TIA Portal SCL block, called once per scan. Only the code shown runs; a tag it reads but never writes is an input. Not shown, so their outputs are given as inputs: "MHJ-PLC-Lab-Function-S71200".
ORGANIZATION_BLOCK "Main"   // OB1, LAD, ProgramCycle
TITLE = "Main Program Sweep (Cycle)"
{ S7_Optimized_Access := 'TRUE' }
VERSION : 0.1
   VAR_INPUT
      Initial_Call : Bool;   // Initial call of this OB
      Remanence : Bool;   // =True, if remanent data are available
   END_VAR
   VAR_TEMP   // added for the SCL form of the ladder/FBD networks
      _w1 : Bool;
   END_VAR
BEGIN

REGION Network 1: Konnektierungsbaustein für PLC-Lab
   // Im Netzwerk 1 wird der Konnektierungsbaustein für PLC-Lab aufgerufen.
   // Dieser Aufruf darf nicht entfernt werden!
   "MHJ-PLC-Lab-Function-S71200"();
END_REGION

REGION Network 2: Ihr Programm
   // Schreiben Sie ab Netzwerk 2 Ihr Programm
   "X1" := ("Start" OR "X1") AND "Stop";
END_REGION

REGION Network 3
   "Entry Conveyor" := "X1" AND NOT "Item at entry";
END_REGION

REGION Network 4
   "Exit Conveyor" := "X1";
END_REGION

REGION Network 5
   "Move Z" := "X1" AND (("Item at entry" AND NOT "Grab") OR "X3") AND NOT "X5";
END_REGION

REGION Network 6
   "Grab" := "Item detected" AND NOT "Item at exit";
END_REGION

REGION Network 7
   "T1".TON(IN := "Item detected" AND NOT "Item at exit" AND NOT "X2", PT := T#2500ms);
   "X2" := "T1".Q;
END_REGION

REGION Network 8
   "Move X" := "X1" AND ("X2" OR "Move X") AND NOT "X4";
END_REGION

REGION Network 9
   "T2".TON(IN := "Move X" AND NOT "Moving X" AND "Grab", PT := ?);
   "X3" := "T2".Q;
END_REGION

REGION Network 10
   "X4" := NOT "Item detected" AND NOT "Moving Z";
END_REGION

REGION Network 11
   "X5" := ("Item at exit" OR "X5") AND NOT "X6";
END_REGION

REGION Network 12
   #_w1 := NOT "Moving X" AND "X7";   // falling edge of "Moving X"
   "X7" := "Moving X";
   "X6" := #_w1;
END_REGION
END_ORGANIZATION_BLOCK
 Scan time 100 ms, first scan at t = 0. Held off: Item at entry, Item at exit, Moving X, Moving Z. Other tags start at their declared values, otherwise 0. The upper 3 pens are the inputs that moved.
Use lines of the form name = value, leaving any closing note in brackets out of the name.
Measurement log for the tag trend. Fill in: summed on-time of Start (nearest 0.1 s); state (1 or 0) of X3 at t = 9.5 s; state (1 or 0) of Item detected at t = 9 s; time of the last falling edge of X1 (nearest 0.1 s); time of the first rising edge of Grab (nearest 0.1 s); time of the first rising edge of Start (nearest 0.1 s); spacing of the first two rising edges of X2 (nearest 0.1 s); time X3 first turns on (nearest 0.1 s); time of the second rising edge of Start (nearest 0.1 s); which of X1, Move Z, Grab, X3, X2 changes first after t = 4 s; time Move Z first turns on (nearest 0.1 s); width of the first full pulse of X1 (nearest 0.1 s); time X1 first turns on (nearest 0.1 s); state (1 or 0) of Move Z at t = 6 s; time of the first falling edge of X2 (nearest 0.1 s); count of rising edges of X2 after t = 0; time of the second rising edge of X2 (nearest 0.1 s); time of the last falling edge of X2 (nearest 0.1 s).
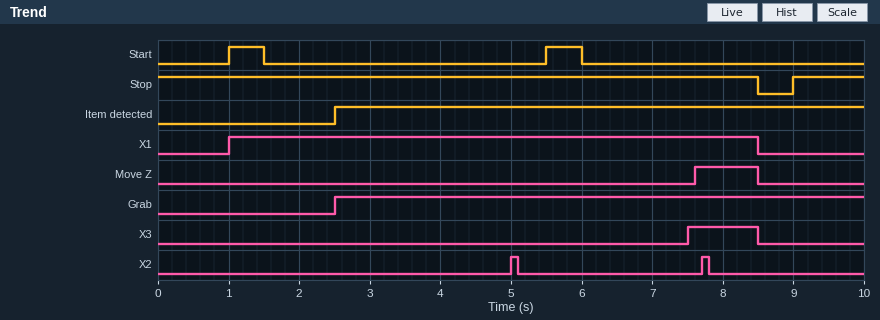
summed on-time of Start = 1.0 s
state (1 or 0) of X3 at t = 9.5 s = 0
state (1 or 0) of Item detected at t = 9 s = 1
time of the last falling edge of X1 = 8.5 s
time of the first rising edge of Grab = 2.5 s
time of the first rising edge of Start = 1.0 s
spacing of the first two rising edges of X2 = 2.7 s
time X3 first turns on = 7.5 s
time of the second rising edge of Start = 5.5 s
which of X1, Move Z, Grab, X3, X2 changes first after t = 4 s = X2
time Move Z first turns on = 7.6 s
width of the first full pulse of X1 = 7.5 s
time X1 first turns on = 1.0 s
state (1 or 0) of Move Z at t = 6 s = 0
time of the first falling edge of X2 = 5.1 s
count of rising edges of X2 after t = 0 = 2
time of the second rising edge of X2 = 7.7 s
time of the last falling edge of X2 = 7.8 s
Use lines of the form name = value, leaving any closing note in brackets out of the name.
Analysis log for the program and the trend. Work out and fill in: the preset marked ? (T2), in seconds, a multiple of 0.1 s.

the preset marked ? (T2), in seconds, a multiple of 0.1 s = 2.5 s
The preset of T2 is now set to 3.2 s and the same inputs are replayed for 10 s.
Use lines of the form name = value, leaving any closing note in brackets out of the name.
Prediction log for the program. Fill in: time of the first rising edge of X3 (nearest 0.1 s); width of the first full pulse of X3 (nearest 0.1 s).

time of the first rising edge of X3 = 8.2 s
width of the first full pulse of X3 = 0.3 s
